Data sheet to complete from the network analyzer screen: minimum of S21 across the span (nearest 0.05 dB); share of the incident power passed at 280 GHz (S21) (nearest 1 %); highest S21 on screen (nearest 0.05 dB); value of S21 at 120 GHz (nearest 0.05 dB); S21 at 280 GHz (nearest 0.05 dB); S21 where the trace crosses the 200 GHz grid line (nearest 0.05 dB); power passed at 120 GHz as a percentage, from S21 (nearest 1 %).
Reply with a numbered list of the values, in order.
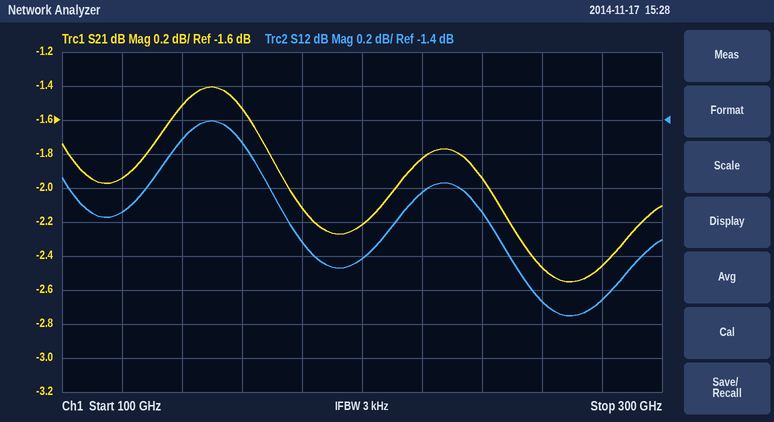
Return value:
1. -2.55 dB
2. 57 %
3. -1.40 dB
4. -1.95 dB
5. -2.45 dB
6. -2.20 dB
7. 64 %
